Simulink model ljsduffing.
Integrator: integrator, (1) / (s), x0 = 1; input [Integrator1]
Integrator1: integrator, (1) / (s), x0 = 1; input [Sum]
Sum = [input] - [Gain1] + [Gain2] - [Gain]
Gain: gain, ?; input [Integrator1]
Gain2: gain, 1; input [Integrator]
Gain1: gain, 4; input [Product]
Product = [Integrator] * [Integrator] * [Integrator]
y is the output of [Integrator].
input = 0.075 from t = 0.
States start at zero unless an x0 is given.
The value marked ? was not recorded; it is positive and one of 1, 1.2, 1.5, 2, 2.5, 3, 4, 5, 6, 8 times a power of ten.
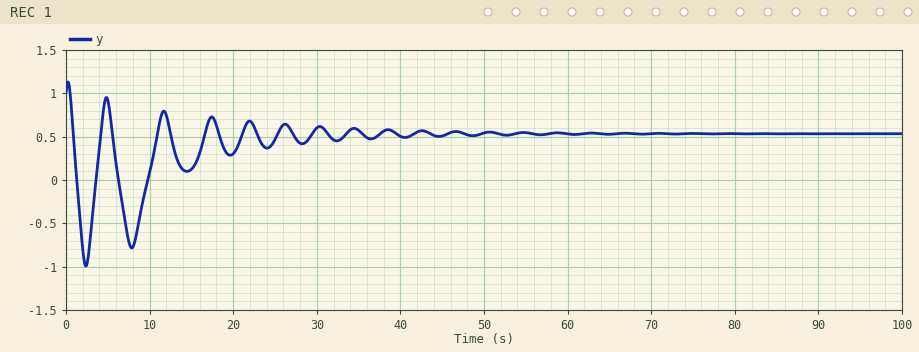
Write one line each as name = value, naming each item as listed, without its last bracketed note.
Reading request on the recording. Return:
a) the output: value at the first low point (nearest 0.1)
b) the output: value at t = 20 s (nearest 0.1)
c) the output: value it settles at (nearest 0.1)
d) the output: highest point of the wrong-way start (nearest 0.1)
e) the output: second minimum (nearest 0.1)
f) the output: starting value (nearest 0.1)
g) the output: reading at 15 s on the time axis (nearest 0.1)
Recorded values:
the output: value at the first low point = -1.0
the output: value at t = 20 s = 0.3
the output: value it settles at = 0.5
the output: highest point of the wrong-way start = 1.1
the output: second minimum = -0.8
the output: starting value = 1.0
the output: reading at 15 s on the time axis = 0.1
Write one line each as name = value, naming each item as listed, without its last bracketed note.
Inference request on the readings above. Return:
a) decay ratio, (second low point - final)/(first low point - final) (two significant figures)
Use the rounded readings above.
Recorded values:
decay ratio, (second low point - final)/(first low point - final) = 0.87
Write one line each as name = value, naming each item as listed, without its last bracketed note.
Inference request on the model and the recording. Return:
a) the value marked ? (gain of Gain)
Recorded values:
the value marked ? = 0.15
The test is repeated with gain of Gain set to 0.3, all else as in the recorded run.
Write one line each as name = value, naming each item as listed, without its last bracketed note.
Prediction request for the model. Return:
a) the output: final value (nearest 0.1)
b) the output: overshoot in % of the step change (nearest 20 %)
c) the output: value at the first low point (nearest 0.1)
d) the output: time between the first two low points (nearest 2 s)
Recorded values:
the output: final value = 0.5
the output: overshoot in % of the step change = 300 %
the output: value at the first low point = -0.9
the output: time between the first two low points = 6 s
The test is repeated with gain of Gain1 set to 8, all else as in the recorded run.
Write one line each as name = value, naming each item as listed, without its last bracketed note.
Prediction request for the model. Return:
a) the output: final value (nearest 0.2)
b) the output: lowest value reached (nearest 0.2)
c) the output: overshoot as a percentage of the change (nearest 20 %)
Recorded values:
the output: final value = 0.4
the output: lowest value reached = -1.0
the output: overshoot as a percentage of the change = 220 %
